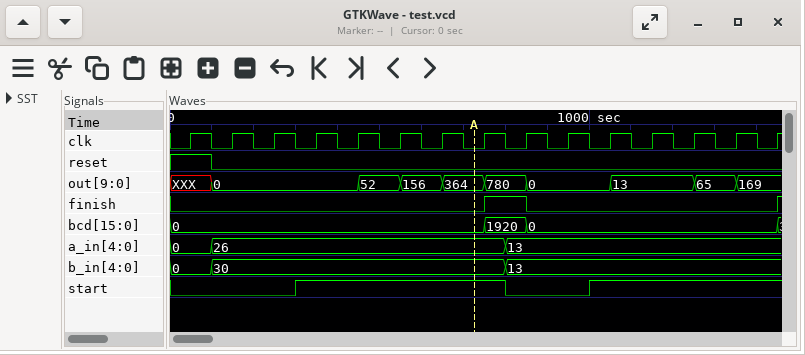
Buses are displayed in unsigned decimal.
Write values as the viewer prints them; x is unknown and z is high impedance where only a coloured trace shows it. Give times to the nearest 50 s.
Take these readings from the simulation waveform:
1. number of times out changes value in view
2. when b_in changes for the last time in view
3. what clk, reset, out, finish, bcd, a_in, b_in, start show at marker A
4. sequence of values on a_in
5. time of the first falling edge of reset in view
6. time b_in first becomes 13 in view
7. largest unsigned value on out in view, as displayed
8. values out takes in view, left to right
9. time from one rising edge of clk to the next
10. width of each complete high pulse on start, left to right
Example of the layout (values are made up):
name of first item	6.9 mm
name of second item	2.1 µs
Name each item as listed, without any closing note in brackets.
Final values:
number of times out changes value in view	9
when b_in changes for the last time in view	800 s
what clk, reset, out, finish, bcd, a_in, b_in, start show at marker A	clk=0, reset=0, out=364, finish=0, bcd=0, a_in=26, b_in=30, start=1
sequence of values on a_in	0, 26, 13
time of the first falling edge of reset in view	100 s
time b_in first becomes 13 in view	800 s
largest unsigned value on out in view, as displayed	780
values out takes in view, left to right	XXX, 0, 52, 156, 364, 780, 0, 13, 65, 169
time from one rising edge of clk to the next	100 s
width of each complete high pulse on start, left to right	500 s
